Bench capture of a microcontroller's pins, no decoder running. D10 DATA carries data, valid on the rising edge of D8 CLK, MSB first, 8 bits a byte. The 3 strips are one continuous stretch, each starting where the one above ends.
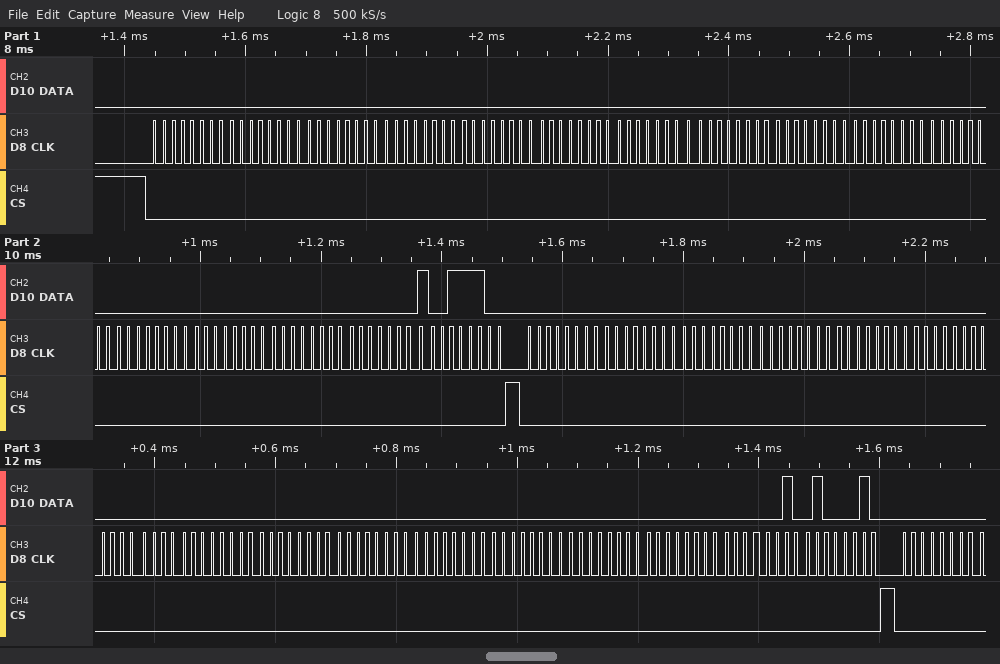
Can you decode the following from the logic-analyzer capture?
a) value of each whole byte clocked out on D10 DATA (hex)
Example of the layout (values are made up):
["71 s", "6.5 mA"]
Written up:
["0x00 0x00 0x00 0x00 0x00 0x00 0x00 0x00 0x00 0x00 0x00 0x00 0x00 0x00 0x01 0x3C 0x00 0x00 0x00 0x00 0x00 0x00 0x00 0x00 0x00 0x00 0x00 0x00 0x00 0x00 0x02 0x42 0x00"]
